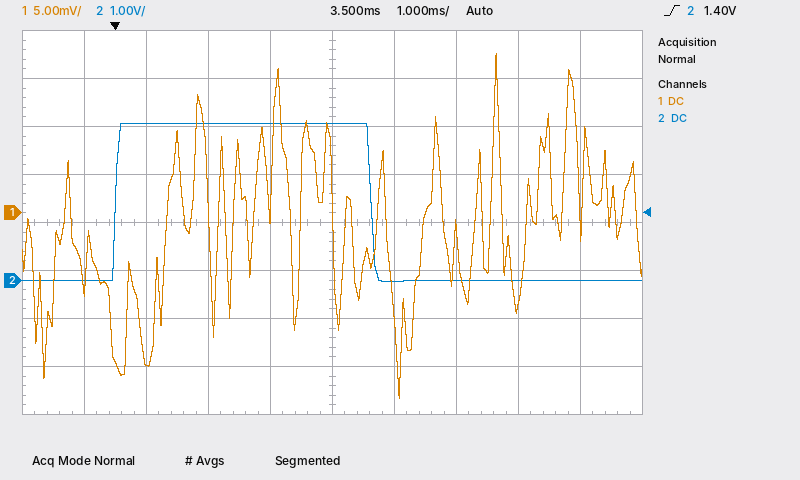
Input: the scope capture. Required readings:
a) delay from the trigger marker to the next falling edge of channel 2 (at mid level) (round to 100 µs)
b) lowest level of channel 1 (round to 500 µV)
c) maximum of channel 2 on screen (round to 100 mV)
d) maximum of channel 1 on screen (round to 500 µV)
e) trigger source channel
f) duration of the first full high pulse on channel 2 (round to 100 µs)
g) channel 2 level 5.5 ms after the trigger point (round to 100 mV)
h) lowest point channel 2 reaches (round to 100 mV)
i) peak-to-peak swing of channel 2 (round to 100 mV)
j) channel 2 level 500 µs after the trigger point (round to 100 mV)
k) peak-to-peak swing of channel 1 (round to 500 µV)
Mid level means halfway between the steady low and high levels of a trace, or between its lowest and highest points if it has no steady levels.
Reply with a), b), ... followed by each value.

a) 4.1 ms
b) -19.5 mV
c) 3.3 V
d) 16.5 mV
e) channel 2
f) 4.1 ms
g) 0.0 V
h) 0.0 V
i) 3.3 V
j) 3.3 V
k) 36.0 mV
